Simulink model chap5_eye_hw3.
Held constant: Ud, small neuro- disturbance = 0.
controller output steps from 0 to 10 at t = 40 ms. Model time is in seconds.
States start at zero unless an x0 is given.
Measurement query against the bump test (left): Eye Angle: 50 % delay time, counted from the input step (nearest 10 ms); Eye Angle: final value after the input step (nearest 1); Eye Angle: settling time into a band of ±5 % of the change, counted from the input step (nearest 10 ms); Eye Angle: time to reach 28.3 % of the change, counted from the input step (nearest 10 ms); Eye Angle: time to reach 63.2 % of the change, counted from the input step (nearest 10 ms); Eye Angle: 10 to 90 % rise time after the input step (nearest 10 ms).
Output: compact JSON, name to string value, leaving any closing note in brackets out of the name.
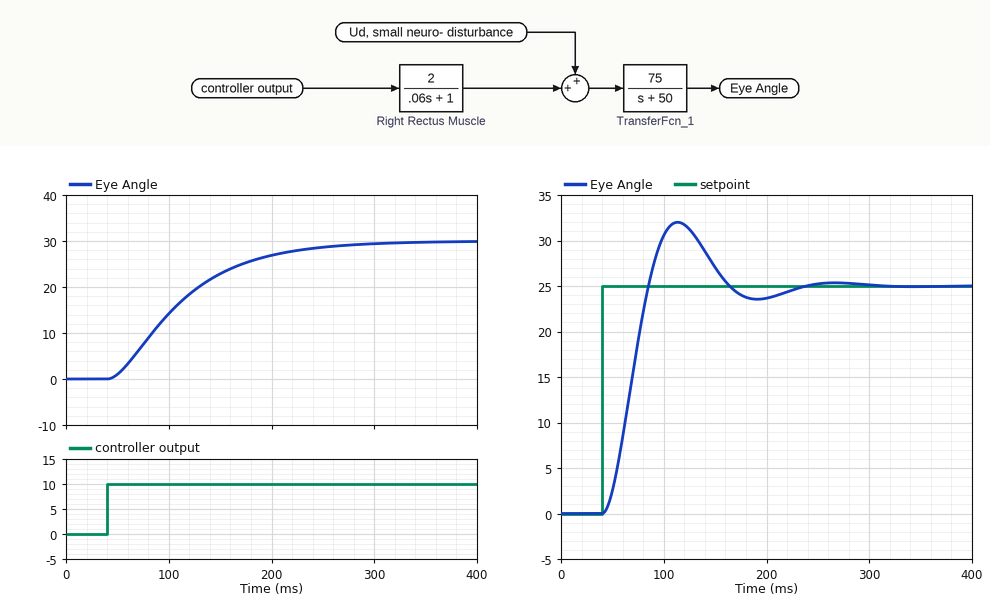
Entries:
{"Eye Angle: 50 % delay time, counted from the input step": "60 ms", "Eye Angle: final value after the input step": "30", "Eye Angle: settling time into a band of ±5 % of the change, counted from the input step": "200 ms", "Eye Angle: time to reach 28.3 % of the change, counted from the input step": "40 ms", "Eye Angle: time to reach 63.2 % of the change, counted from the input step": "80 ms", "Eye Angle: 10 to 90 % rise time after the input step": "140 ms"}
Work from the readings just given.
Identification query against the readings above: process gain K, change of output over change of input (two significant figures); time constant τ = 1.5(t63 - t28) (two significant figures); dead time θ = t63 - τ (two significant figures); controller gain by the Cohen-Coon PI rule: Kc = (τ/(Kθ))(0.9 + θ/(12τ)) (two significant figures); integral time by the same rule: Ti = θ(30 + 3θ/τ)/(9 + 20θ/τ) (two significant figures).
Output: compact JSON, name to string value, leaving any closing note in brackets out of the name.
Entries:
{"process gain K, change of output over change of input": "3.0", "time constant τ = 1.5(t63 - t28)": "60 ms", "dead time θ = t63 - τ": "20 ms", "controller gain by the Cohen-Coon PI rule: Kc = (τ/(Kθ))(0.9 + θ/(12τ))": "0.93", "integral time by the same rule: Ti = θ(30 + 3θ/τ)/(9 + 20θ/τ)": "40 ms"}
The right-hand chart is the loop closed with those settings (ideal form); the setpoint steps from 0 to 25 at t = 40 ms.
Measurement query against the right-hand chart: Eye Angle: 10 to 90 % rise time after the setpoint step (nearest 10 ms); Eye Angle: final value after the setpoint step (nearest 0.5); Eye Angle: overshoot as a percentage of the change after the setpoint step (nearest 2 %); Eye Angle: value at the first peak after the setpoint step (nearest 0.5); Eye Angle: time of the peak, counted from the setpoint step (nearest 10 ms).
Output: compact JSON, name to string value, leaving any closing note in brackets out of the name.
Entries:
{"Eye Angle: 10 to 90 % rise time after the setpoint step": "30 ms", "Eye Angle: final value after the setpoint step": "25.0", "Eye Angle: overshoot as a percentage of the change after the setpoint step": "28 %", "Eye Angle: value at the first peak after the setpoint step": "32.0", "Eye Angle: time of the peak, counted from the setpoint step": "70 ms"}
